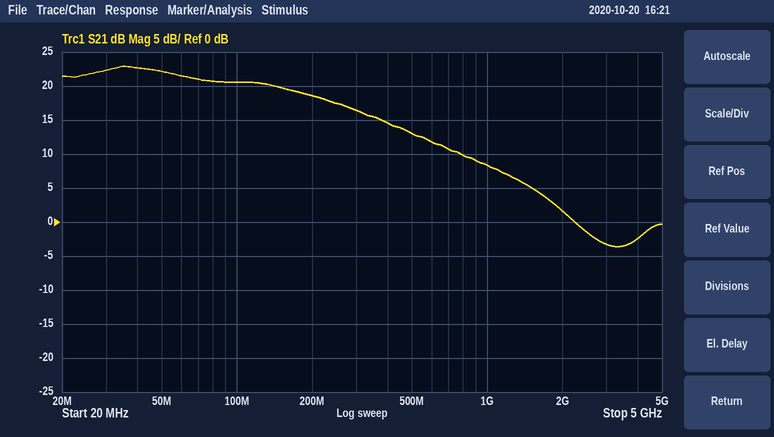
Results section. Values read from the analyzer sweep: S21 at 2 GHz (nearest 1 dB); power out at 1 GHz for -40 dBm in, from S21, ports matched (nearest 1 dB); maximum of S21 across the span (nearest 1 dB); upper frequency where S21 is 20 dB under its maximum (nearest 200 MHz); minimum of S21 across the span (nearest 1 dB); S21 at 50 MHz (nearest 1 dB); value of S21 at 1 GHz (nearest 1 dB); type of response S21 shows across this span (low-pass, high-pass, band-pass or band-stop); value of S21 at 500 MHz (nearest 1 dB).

2 dB
-32 dBm
23 dB
1.8 GHz
-4 dB
22 dB
8 dB
low-pass
13 dB
